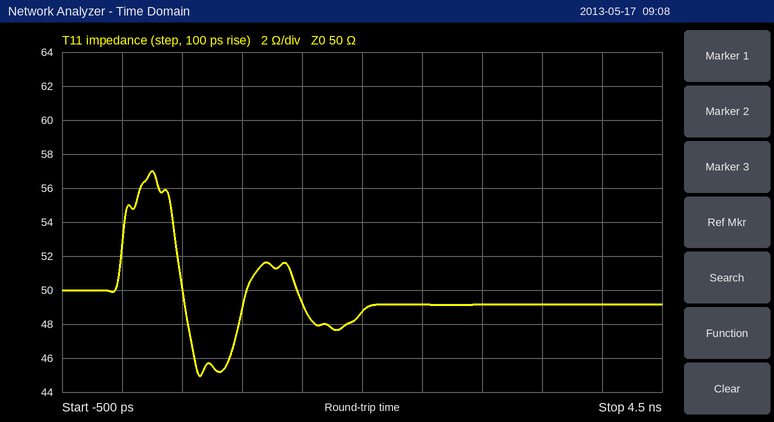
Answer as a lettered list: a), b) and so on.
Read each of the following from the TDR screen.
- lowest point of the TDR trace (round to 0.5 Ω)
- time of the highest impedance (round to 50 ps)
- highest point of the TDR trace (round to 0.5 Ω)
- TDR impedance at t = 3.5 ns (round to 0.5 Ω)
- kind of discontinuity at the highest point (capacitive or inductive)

a) 45.0 Ω
b) 250 ps
c) 57.0 Ω
d) 49.0 Ω
e) inductive
